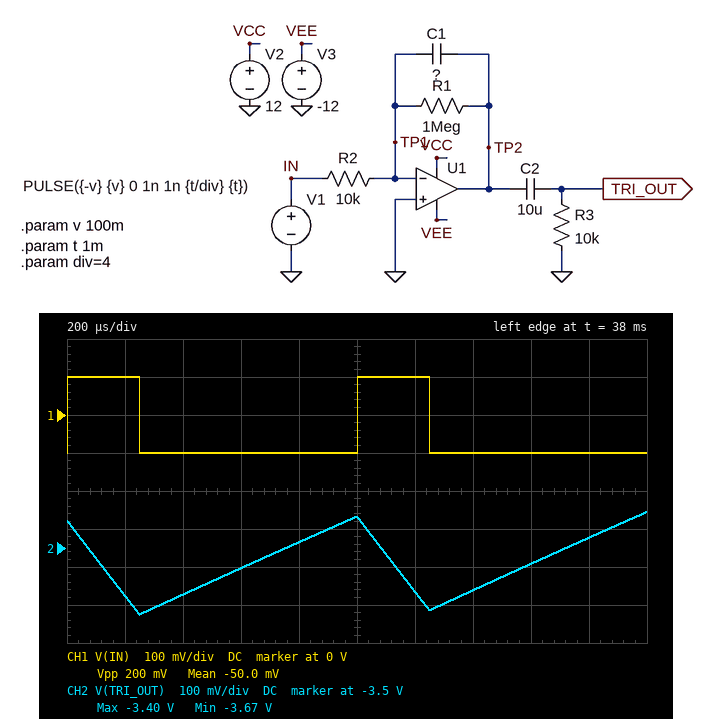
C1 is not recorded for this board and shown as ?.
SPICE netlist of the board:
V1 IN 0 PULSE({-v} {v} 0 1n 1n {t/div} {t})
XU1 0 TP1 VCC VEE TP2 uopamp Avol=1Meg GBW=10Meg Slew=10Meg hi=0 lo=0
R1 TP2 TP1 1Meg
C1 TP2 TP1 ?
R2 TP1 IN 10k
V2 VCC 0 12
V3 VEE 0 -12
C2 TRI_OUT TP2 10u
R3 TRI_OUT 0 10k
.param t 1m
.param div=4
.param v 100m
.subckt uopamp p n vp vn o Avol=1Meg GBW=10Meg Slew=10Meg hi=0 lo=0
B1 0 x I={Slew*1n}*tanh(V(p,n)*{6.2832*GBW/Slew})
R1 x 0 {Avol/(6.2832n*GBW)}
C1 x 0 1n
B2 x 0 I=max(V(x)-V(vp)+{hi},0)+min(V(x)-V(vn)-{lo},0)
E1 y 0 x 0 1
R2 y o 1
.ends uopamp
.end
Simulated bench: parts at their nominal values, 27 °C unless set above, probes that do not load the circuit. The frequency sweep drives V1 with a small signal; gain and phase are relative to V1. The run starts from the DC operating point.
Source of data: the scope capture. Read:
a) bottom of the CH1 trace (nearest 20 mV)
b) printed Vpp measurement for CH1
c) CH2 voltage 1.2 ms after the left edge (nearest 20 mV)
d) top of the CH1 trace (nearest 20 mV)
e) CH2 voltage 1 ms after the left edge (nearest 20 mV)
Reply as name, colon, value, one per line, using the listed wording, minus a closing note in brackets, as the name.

bottom of the CH1 trace: -100 mV
printed Vpp measurement for CH1: 200 mV
CH2 voltage 1.2 ms after the left edge: -3.62 V
top of the CH1 trace: 100 mV
CH2 voltage 1 ms after the left edge: -3.42 V
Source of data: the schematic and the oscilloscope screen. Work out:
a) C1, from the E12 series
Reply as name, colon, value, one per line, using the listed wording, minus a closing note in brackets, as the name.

C1, from the E12 series: 15 nF
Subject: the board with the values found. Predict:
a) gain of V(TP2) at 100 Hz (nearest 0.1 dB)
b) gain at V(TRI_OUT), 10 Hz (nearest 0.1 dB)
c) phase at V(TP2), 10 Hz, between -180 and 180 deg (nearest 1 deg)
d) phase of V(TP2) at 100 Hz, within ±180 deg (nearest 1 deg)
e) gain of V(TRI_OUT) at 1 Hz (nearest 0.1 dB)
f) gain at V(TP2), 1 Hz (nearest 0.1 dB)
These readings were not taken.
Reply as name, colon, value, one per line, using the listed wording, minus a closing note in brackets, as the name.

gain of V(TP2) at 100 Hz: 20.5 dB
gain at V(TRI_OUT), 10 Hz: 37.1 dB
phase at V(TP2), 10 Hz, between -180 and 180 deg: 137 deg
phase of V(TP2) at 100 Hz, within ±180 deg: 96 deg
gain of V(TRI_OUT) at 1 Hz: 34.5 dB
gain at V(TP2), 1 Hz: 40.0 dB
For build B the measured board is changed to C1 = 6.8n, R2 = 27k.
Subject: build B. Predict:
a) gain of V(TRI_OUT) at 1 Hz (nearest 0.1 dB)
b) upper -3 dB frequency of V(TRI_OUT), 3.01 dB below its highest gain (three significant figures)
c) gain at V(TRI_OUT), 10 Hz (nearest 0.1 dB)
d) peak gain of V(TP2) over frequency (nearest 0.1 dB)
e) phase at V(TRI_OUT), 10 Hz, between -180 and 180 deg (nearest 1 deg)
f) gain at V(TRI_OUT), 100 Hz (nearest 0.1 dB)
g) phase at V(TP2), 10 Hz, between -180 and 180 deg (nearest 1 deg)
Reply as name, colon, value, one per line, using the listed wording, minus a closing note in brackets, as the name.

gain of V(TRI_OUT) at 1 Hz: 25.9 dB
upper -3 dB frequency of V(TRI_OUT), 3.01 dB below its highest gain: 26.4 Hz
gain at V(TRI_OUT), 10 Hz: 30.5 dB
peak gain of V(TP2) over frequency: 31.4 dB
phase at V(TRI_OUT), 10 Hz, between -180 and 180 deg: 166 deg
gain at V(TRI_OUT), 100 Hz: 18.5 dB
phase at V(TP2), 10 Hz, between -180 and 180 deg: 157 deg
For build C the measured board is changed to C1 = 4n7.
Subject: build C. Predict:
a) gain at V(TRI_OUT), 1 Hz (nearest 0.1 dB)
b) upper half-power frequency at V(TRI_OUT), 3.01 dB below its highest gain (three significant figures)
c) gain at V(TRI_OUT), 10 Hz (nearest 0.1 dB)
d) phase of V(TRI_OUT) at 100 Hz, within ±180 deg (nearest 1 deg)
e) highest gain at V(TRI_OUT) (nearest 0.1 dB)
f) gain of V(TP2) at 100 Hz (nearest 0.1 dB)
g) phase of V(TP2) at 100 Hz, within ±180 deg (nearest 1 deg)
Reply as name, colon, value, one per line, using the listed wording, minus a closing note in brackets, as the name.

gain at V(TRI_OUT), 1 Hz: 34.5 dB
upper half-power frequency at V(TRI_OUT), 3.01 dB below its highest gain: 36.9 Hz
gain at V(TRI_OUT), 10 Hz: 39.5 dB
phase of V(TRI_OUT) at 100 Hz, within ±180 deg: 110 deg
highest gain at V(TRI_OUT): 39.6 dB
gain of V(TP2) at 100 Hz: 30.1 dB
phase of V(TP2) at 100 Hz, within ±180 deg: 109 deg
